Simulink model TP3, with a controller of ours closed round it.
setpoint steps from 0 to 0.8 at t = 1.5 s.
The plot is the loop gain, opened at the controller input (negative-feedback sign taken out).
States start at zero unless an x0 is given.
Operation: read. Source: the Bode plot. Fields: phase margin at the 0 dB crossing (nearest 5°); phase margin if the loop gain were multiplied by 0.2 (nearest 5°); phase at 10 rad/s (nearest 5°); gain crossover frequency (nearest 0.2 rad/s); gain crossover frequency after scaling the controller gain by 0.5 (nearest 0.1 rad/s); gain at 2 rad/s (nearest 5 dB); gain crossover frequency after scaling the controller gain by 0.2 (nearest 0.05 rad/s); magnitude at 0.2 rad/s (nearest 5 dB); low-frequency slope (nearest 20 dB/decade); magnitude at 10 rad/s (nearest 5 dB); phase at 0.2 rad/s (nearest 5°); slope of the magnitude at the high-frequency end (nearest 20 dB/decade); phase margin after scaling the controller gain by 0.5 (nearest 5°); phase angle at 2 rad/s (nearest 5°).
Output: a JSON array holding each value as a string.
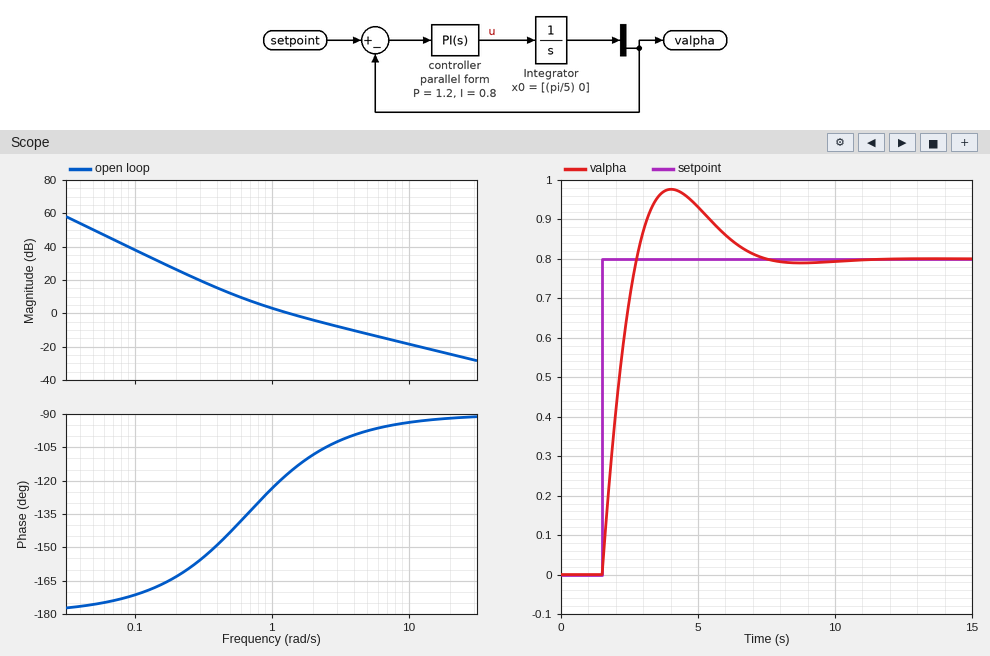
["65°", "35°", "-95°", "1.4 rad/s", "0.8 rad/s", "-5 dB", "0.45 rad/s", "25 dB", "-40 dB/decade", "-20 dB", "-165°", "-20 dB/decade", "50°", "-110°"]
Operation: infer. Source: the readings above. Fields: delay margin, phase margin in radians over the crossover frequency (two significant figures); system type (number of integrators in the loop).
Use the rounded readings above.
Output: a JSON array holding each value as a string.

["0.81 s", "2"]
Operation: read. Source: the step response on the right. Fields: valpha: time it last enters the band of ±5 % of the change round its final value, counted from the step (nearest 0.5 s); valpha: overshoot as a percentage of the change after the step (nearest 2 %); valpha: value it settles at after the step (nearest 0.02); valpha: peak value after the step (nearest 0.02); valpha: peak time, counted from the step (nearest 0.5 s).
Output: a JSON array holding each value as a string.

["5.0 s", "22 %", "0.80", "0.98", "2.5 s"]
